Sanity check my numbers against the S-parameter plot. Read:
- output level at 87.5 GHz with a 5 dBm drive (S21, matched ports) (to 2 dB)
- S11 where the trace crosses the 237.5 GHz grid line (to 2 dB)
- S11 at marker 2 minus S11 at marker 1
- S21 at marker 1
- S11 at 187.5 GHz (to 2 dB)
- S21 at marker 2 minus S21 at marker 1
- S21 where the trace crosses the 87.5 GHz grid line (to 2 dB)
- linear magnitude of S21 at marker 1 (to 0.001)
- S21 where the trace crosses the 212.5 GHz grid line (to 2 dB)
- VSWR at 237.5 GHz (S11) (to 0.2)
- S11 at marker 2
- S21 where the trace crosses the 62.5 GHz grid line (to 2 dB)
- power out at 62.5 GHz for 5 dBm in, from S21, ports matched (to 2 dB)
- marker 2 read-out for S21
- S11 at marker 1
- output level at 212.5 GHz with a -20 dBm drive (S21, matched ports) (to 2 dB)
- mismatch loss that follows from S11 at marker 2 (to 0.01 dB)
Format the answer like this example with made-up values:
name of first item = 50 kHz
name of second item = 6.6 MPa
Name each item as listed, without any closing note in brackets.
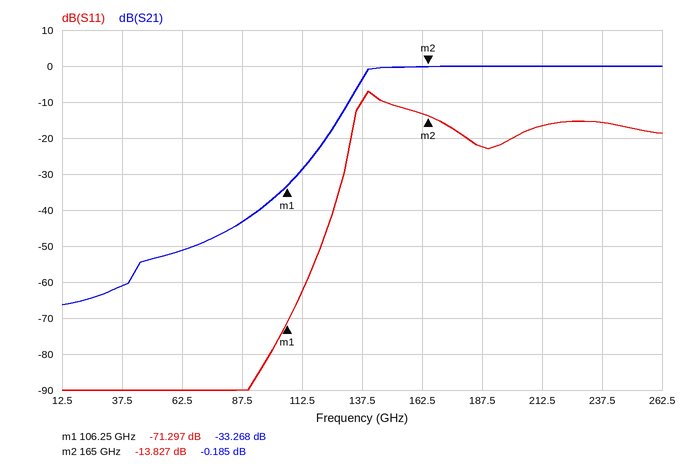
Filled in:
output level at 87.5 GHz with a 5 dBm drive (S21, matched ports) = -38 dBm
S11 where the trace crosses the 237.5 GHz grid line = -16 dB
S11 at marker 2 minus S11 at marker 1 = 57.470 dB
S21 at marker 1 = -33.268 dB
S11 at 187.5 GHz = -22 dB
S21 at marker 2 minus S21 at marker 1 = 33.083 dB
S21 where the trace crosses the 87.5 GHz grid line = -44 dB
linear magnitude of S21 at marker 1 = 0.022
S21 where the trace crosses the 212.5 GHz grid line = 0 dB
VSWR at 237.5 GHz (S11) = 1.4
S11 at marker 2 = -13.827 dB
S21 where the trace crosses the 62.5 GHz grid line = -52 dB
power out at 62.5 GHz for 5 dBm in, from S21, ports matched = -46 dBm
marker 2 read-out for S21 = -0.185 dB
S11 at marker 1 = -71.297 dB
output level at 212.5 GHz with a -20 dBm drive (S21, matched ports) = -20 dBm
mismatch loss that follows from S11 at marker 2 = 0.18 dB
